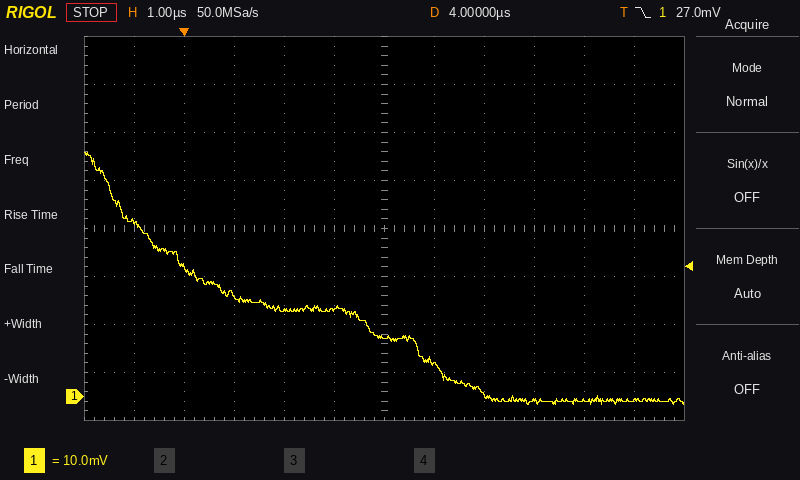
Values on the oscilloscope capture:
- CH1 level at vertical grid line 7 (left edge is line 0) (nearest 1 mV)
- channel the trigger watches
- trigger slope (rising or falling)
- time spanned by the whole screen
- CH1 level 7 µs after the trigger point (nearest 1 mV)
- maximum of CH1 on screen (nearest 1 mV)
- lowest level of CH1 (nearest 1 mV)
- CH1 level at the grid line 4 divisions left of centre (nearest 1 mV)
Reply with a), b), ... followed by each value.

a) 7 mV
b) CH1
c) falling
d) 12 µs
e) -1 mV
f) 51 mV
g) -2 mV
h) 27 mV
